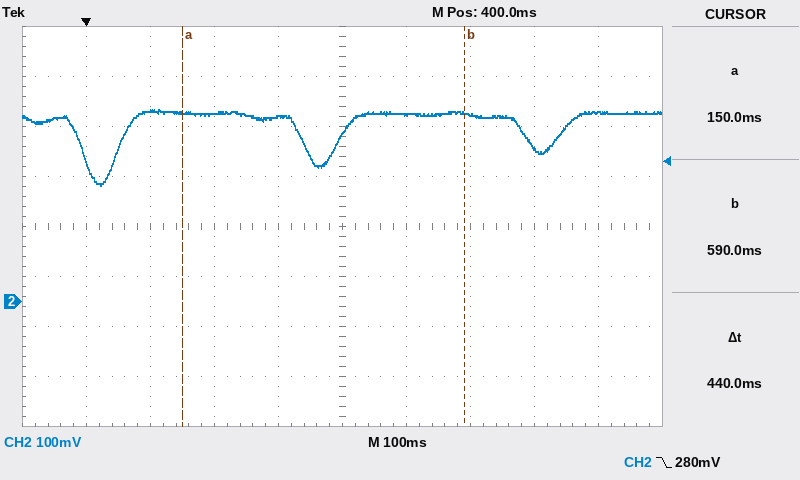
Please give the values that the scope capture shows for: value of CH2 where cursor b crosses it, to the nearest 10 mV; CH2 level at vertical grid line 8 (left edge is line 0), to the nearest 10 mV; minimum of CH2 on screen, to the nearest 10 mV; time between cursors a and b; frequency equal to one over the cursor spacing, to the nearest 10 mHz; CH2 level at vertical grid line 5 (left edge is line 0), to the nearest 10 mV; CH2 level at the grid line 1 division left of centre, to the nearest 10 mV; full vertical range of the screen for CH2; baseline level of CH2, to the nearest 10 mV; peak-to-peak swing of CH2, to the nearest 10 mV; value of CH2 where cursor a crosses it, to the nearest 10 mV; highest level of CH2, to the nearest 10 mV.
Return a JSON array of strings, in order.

["380 mV", "310 mV", "230 mV", "440 ms", "2.27 Hz", "330 mV", "370 mV", "800 mV", "380 mV", "150 mV", "380 mV", "380 mV"]
